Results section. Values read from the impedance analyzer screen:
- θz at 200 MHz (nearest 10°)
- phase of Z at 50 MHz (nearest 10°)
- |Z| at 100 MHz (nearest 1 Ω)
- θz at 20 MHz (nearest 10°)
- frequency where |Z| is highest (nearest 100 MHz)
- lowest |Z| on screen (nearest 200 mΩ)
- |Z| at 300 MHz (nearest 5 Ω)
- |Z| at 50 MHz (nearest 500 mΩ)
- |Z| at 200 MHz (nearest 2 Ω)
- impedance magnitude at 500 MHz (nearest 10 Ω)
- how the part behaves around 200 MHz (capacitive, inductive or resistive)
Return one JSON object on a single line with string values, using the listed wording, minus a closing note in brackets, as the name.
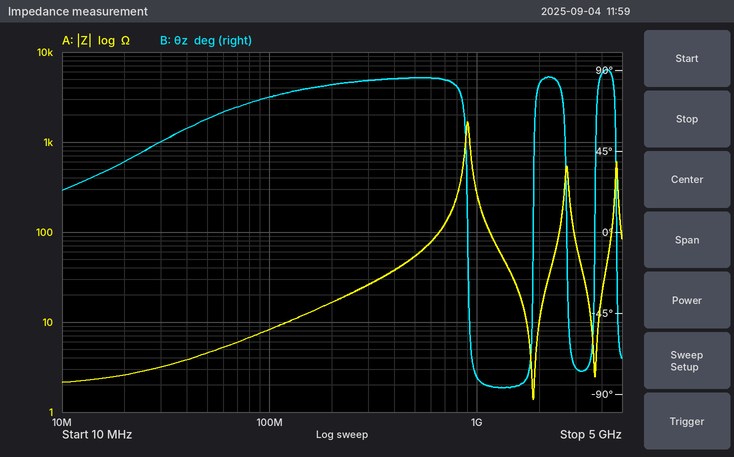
{"θz at 200 MHz": "80°", "phase of Z at 50 MHz": "60°", "|Z| at 100 MHz": "8 Ω", "θz at 20 MHz": "40°", "frequency where |Z| is highest": "900 MHz", "lowest |Z| on screen": "1.4 Ω", "|Z| at 300 MHz": "25 Ω", "|Z| at 50 MHz": "4.5 Ω", "|Z| at 200 MHz": "16 Ω", "impedance magnitude at 500 MHz": "50 Ω", "how the part behaves around 200 MHz": "inductive"}
